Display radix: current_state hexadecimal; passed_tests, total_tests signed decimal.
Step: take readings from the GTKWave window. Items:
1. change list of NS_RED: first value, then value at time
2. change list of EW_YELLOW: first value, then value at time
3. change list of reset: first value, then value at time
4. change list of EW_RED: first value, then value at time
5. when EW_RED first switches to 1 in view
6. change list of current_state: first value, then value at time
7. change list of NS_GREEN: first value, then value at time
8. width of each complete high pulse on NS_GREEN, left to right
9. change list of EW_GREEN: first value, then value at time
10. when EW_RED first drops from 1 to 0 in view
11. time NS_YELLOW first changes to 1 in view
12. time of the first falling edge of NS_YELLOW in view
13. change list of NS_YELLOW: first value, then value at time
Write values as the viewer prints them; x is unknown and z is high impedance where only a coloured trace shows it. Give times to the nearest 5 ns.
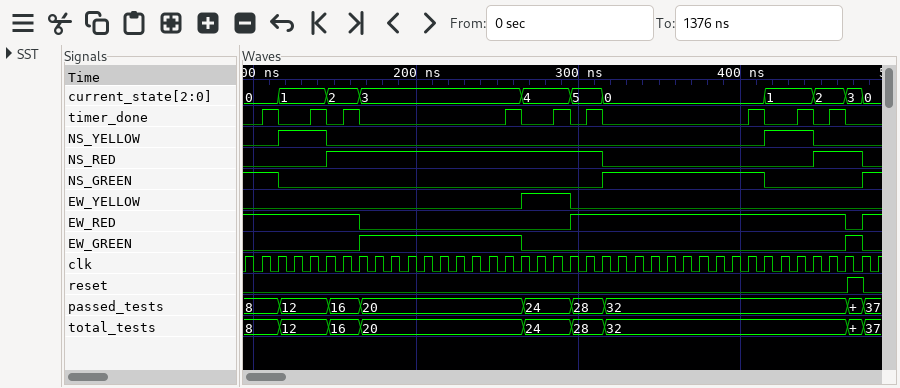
0, 1 at 145 ns, 0 at 315 ns, 1 at 445 ns, 0 at 475 ns
0, 1 at 265 ns, 0 at 295 ns
0, 1 at 465 ns, 0 at 475 ns
1, 0 at 165 ns, 1 at 295 ns, 0 at 465 ns, 1 at 475 ns
295 ns
0, 1 at 115 ns, 2 at 145 ns, 3 at 165 ns, 4 at 265 ns, 5 at 295 ns, 0 at 315 ns, 1 at 415 ns, 2 at 445 ns, 3 at 465 ns, 0 at 475 ns
1, 0 at 115 ns, 1 at 315 ns, 0 at 415 ns, 1 at 475 ns
100 ns
0, 1 at 165 ns, 0 at 265 ns, 1 at 465 ns, 0 at 475 ns
165 ns
115 ns
145 ns
0, 1 at 115 ns, 0 at 145 ns, 1 at 415 ns, 0 at 445 ns
